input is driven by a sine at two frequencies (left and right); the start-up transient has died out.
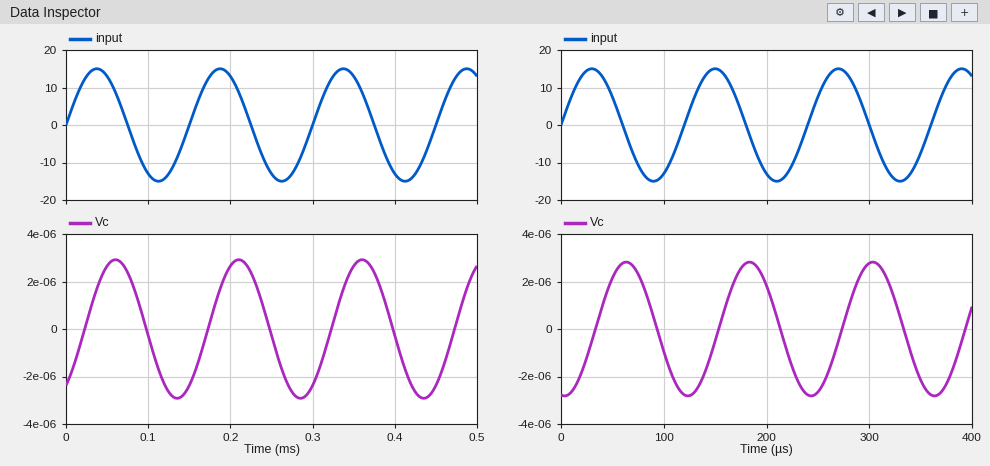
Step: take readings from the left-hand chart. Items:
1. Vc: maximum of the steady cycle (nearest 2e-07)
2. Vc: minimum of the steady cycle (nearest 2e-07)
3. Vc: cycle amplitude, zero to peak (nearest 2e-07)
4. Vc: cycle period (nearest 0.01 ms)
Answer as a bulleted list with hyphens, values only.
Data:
- 0.0000030
- -0.0000030
- 0.0000030
- 0.15 ms
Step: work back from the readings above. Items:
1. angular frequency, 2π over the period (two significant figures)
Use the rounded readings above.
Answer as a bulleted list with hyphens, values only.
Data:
- 42 rad/ms
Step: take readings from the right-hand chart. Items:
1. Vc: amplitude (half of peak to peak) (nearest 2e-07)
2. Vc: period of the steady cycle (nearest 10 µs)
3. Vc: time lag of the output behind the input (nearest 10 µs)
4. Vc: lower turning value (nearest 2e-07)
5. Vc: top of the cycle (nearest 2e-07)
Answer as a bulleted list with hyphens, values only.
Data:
- 0.0000028
- 120 µs
- 30 µs
- -0.0000028
- 0.0000028
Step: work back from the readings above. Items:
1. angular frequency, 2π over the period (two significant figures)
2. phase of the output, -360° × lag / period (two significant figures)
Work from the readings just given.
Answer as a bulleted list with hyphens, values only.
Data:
- 0.052 rad/µs
- -90°
